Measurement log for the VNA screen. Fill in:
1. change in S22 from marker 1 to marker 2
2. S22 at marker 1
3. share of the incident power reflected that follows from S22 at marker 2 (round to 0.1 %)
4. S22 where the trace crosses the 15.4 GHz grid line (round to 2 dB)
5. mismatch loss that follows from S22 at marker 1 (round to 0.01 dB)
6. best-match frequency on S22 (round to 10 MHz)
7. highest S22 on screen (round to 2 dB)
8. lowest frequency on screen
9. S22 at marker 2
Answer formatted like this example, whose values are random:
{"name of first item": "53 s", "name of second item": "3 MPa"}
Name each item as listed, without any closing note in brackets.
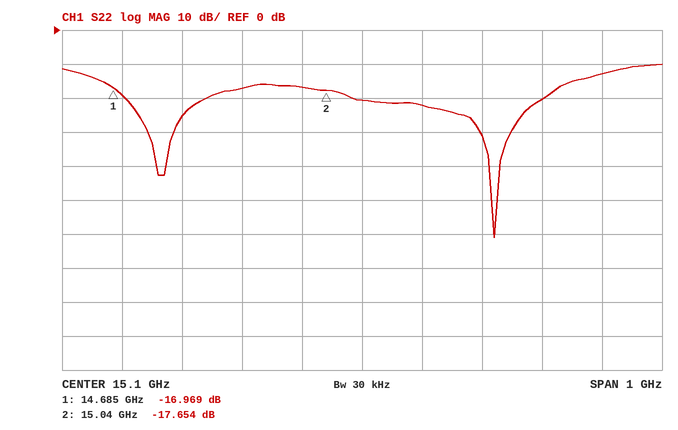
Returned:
{"change in S22 from marker 1 to marker 2": "-0.685 dB", "S22 at marker 1": "-16.969 dB", "share of the incident power reflected that follows from S22 at marker 2": "1.7 %", "S22 where the trace crosses the 15.4 GHz grid line": "-20 dB", "mismatch loss that follows from S22 at marker 1": "0.09 dB", "best-match frequency on S22": "15.32 GHz", "highest S22 on screen": "-10 dB", "lowest frequency on screen": "14.6 GHz", "S22 at marker 2": "-17.654 dB"}
